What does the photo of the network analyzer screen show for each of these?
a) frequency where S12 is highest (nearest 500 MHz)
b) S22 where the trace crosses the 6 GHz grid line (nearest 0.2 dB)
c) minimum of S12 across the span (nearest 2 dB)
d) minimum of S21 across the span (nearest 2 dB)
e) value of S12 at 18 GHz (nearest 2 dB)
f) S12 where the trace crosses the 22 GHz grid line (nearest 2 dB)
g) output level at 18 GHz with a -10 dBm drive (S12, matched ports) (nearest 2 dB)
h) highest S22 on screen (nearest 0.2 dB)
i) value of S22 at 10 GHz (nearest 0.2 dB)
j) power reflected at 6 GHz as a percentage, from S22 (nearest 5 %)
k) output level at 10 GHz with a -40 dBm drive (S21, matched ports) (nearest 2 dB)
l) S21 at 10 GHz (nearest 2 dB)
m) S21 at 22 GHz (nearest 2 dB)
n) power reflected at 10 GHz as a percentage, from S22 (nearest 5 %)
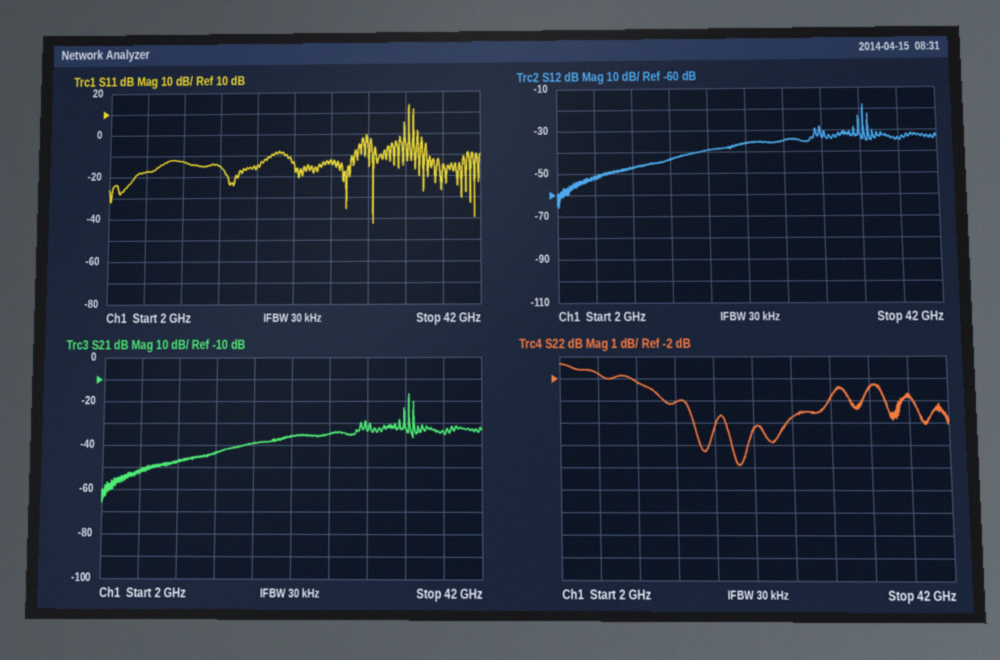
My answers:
34.5 GHz
-1.8 dB
-66 dB
-66 dB
-40 dB
-36 dB
-50 dBm
-1.4 dB
-2.2 dB
65 %
-88 dBm
-48 dB
-36 dB
60 %
